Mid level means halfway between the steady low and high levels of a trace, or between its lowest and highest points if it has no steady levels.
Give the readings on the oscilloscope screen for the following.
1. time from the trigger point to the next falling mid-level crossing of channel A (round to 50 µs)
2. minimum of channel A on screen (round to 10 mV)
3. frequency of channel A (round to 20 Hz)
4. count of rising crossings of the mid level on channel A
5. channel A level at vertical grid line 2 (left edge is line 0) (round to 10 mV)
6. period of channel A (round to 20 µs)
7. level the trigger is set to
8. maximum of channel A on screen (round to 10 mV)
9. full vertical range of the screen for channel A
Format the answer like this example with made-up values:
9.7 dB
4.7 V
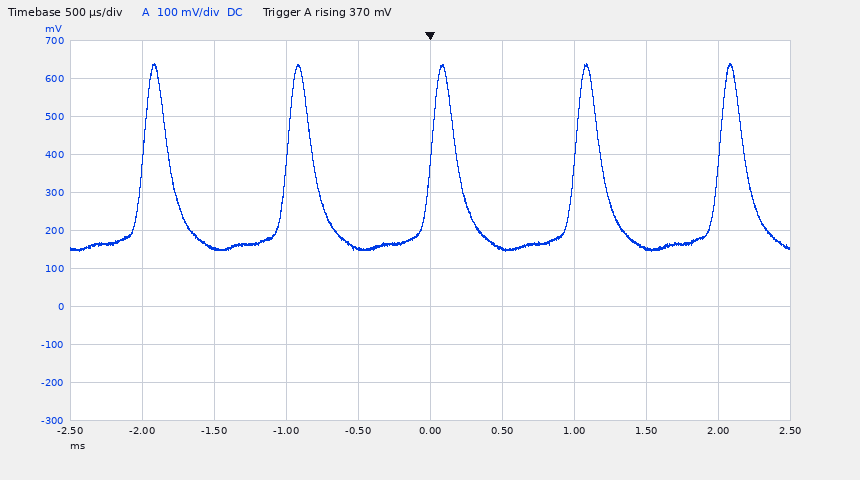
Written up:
200 µs
140 mV
1.00 kHz
5
150 mV
1.00 ms
370 mV
640 mV
1 V
